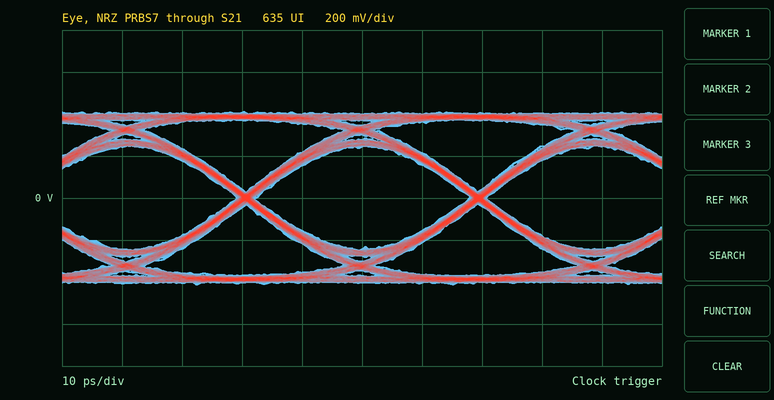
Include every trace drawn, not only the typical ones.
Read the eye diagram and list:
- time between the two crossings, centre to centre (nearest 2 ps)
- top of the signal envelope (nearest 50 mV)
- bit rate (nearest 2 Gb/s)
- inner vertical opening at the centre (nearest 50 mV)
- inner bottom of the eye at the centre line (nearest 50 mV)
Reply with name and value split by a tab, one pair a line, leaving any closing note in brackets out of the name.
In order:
time between the two crossings, centre to centre	38 ps
top of the signal envelope	400 mV
bit rate	26 Gb/s
inner vertical opening at the centre	500 mV
inner bottom of the eye at the centre line	-250 mV
